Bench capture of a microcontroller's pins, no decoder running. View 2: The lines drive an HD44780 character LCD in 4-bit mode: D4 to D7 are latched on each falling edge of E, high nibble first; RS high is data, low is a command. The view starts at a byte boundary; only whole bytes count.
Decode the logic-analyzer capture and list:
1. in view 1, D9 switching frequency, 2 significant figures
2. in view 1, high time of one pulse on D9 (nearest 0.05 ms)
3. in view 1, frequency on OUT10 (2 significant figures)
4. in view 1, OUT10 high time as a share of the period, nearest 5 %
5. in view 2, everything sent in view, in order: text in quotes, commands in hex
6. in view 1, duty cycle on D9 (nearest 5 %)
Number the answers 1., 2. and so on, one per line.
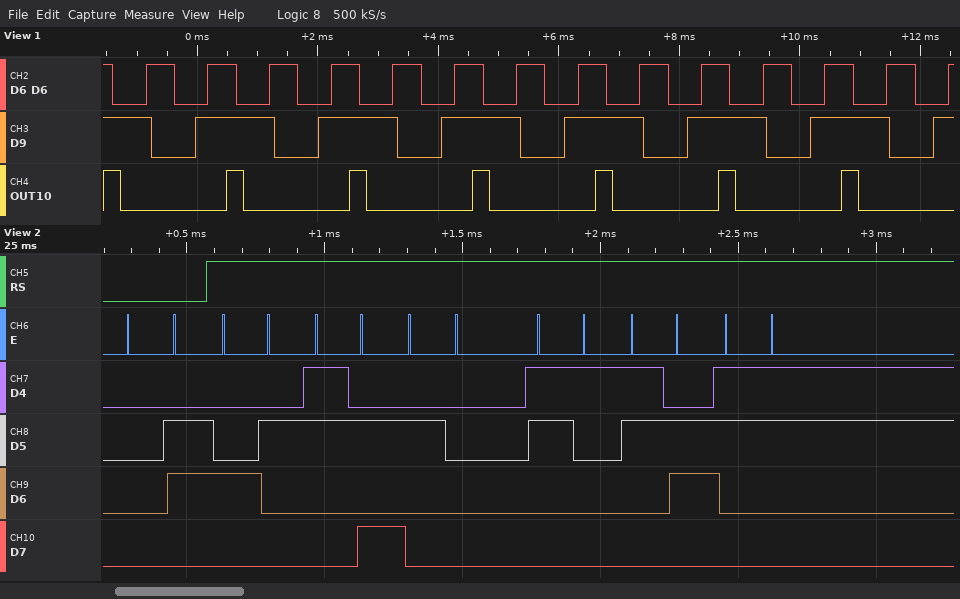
1. 490 Hz
2. 1.30 ms
3. 490 Hz
4. 15 %
5. 0x06 "B: 163"
6. 65 %
